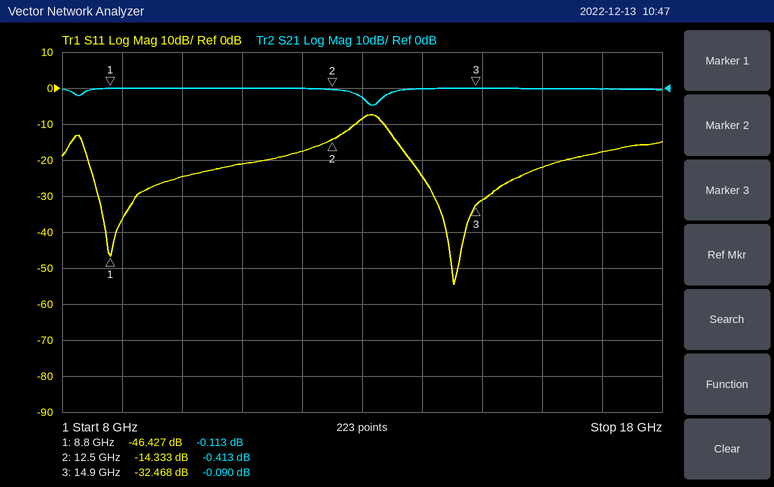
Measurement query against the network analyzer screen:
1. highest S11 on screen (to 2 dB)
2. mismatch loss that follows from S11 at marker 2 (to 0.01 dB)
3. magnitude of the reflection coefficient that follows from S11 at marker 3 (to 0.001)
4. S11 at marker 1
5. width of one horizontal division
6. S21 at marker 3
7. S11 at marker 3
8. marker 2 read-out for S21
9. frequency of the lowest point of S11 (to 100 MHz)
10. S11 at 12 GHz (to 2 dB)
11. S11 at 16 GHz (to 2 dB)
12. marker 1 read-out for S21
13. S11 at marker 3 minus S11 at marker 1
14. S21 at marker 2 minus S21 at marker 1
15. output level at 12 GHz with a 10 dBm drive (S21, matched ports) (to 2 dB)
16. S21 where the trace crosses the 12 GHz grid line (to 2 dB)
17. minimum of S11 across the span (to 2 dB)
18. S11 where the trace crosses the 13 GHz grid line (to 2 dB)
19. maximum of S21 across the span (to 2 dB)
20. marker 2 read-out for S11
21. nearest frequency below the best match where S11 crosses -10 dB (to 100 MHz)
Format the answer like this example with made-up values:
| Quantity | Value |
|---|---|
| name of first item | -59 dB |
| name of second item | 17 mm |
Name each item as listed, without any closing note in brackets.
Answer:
| Quantity | Value |
|---|---|
| highest S11 on screen | -8 dB |
| mismatch loss that follows from S11 at marker 2 | 0.16 dB |
| magnitude of the reflection coefficient that follows from S11 at marker 3 | 0.024 |
| S11 at marker 1 | -46.427 dB |
| width of one horizontal division | 1 GHz |
| S21 at marker 3 | -0.090 dB |
| S11 at marker 3 | -32.468 dB |
| marker 2 read-out for S21 | -0.413 dB |
| frequency of the lowest point of S11 | 14.5 GHz |
| S11 at 12 GHz | -18 dB |
| S11 at 16 GHz | -22 dB |
| marker 1 read-out for S21 | -0.113 dB |
| S11 at marker 3 minus S11 at marker 1 | 13.959 dB |
| S21 at marker 2 minus S21 at marker 1 | -0.300 dB |
| output level at 12 GHz with a 10 dBm drive (S21, matched ports) | 10 dBm |
| S21 where the trace crosses the 12 GHz grid line | 0 dB |
| minimum of S11 across the span | -54 dB |
| S11 where the trace crosses the 13 GHz grid line | -8 dB |
| maximum of S21 across the span | 0 dB |
| marker 2 read-out for S11 | -14.333 dB |
| nearest frequency below the best match where S11 crosses -10 dB | 13.4 GHz |
